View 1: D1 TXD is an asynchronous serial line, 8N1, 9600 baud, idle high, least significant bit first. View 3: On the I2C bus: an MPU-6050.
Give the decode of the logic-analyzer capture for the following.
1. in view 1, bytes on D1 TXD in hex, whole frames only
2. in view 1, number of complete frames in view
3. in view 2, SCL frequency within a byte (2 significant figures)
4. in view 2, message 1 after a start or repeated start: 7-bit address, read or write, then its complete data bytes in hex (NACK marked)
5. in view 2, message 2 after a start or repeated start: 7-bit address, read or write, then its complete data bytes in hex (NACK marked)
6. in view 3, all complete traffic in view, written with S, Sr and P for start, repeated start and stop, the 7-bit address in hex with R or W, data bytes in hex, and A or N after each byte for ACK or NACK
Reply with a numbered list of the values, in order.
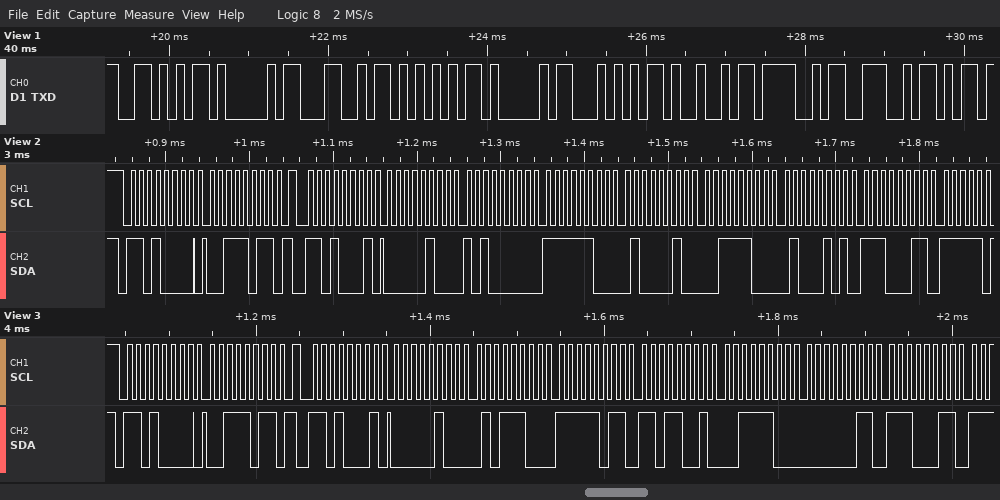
1. 56 41 4C 55 41 54 49 4F 4E
2. 9
3. 100 kHz
4. 0x68 write: 3B
5. 0x68 read: 04 A0 FC 42 3C 45 E3
6. S 68W A 3B A Sr 68R A 04 A 5C A FB A D9 A 3C A 03 A E3 A
